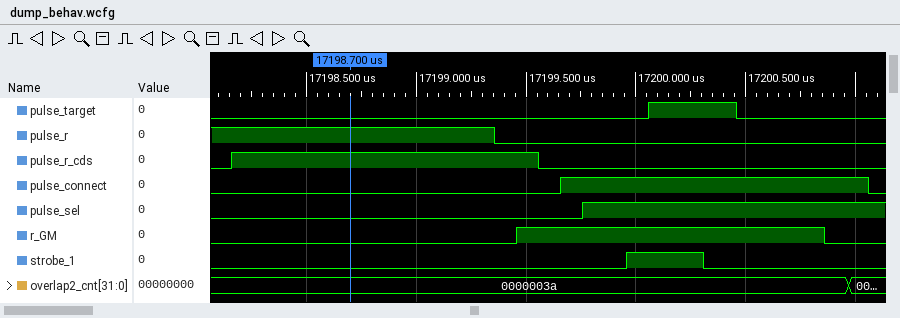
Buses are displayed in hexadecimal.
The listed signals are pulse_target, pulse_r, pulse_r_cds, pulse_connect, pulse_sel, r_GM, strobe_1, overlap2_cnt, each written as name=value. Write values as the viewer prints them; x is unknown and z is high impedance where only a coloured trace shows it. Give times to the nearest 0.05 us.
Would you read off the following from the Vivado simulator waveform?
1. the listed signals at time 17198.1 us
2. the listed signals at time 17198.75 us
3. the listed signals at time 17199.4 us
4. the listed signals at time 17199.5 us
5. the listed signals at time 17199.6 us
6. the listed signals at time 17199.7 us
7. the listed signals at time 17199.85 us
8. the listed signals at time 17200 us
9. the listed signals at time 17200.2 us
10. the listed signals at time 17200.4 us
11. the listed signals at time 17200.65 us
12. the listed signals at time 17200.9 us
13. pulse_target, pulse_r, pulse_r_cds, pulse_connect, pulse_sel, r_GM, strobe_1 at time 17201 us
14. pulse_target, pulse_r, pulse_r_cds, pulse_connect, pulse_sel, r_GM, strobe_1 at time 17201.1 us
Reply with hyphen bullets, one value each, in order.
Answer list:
- pulse_target=0, pulse_r=1, pulse_r_cds=0, pulse_connect=0, pulse_sel=0, r_GM=0, strobe_1=0, overlap2_cnt=0000003a
- pulse_target=0, pulse_r=1, pulse_r_cds=1, pulse_connect=0, pulse_sel=0, r_GM=0, strobe_1=0, overlap2_cnt=0000003a
- pulse_target=0, pulse_r=0, pulse_r_cds=1, pulse_connect=0, pulse_sel=0, r_GM=0, strobe_1=0, overlap2_cnt=0000003a
- pulse_target=0, pulse_r=0, pulse_r_cds=1, pulse_connect=0, pulse_sel=0, r_GM=1, strobe_1=0, overlap2_cnt=0000003a
- pulse_target=0, pulse_r=0, pulse_r_cds=0, pulse_connect=0, pulse_sel=0, r_GM=1, strobe_1=0, overlap2_cnt=0000003a
- pulse_target=0, pulse_r=0, pulse_r_cds=0, pulse_connect=1, pulse_sel=0, r_GM=1, strobe_1=0, overlap2_cnt=0000003a
- pulse_target=0, pulse_r=0, pulse_r_cds=0, pulse_connect=1, pulse_sel=1, r_GM=1, strobe_1=0, overlap2_cnt=0000003a
- pulse_target=0, pulse_r=0, pulse_r_cds=0, pulse_connect=1, pulse_sel=1, r_GM=1, strobe_1=1, overlap2_cnt=0000003a
- pulse_target=1, pulse_r=0, pulse_r_cds=0, pulse_connect=1, pulse_sel=1, r_GM=1, strobe_1=1, overlap2_cnt=0000003a
- pulse_target=1, pulse_r=0, pulse_r_cds=0, pulse_connect=1, pulse_sel=1, r_GM=1, strobe_1=0, overlap2_cnt=0000003a
- pulse_target=0, pulse_r=0, pulse_r_cds=0, pulse_connect=1, pulse_sel=1, r_GM=1, strobe_1=0, overlap2_cnt=0000003a
- pulse_target=0, pulse_r=0, pulse_r_cds=0, pulse_connect=1, pulse_sel=1, r_GM=0, strobe_1=0, overlap2_cnt=0000003a
- pulse_target=0, pulse_r=0, pulse_r_cds=0, pulse_connect=1, pulse_sel=1, r_GM=0, strobe_1=0
- pulse_target=0, pulse_r=0, pulse_r_cds=0, pulse_connect=0, pulse_sel=1, r_GM=0, strobe_1=0
